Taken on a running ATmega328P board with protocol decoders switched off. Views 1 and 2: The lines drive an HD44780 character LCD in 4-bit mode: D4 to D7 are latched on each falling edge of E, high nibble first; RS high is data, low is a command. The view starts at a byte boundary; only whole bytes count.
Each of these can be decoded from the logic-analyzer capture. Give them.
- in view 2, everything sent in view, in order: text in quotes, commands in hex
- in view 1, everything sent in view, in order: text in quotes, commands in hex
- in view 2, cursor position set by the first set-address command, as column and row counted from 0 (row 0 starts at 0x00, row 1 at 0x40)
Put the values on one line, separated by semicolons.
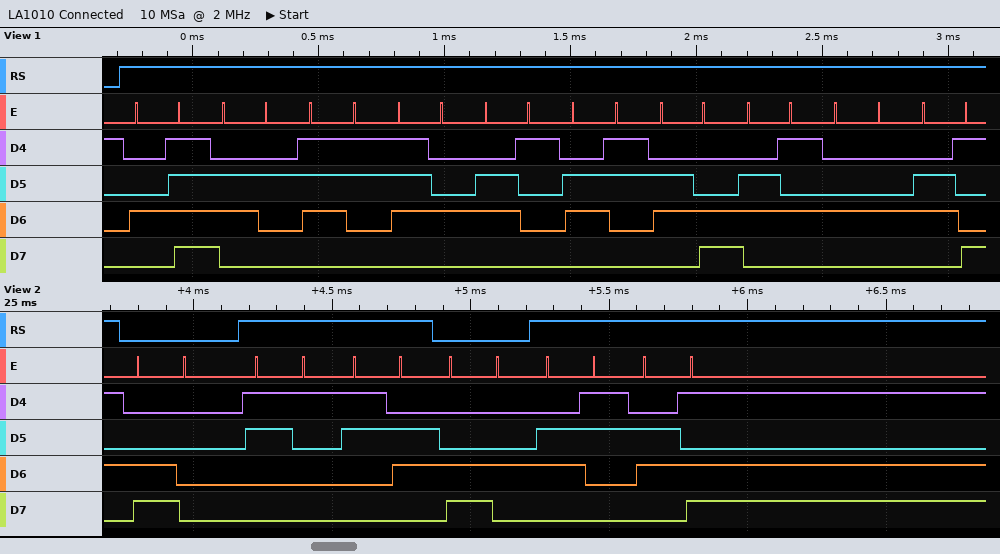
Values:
0xC0 "16" 0xC4 "cm"; "ObstacleDi"; column 0, row 1
